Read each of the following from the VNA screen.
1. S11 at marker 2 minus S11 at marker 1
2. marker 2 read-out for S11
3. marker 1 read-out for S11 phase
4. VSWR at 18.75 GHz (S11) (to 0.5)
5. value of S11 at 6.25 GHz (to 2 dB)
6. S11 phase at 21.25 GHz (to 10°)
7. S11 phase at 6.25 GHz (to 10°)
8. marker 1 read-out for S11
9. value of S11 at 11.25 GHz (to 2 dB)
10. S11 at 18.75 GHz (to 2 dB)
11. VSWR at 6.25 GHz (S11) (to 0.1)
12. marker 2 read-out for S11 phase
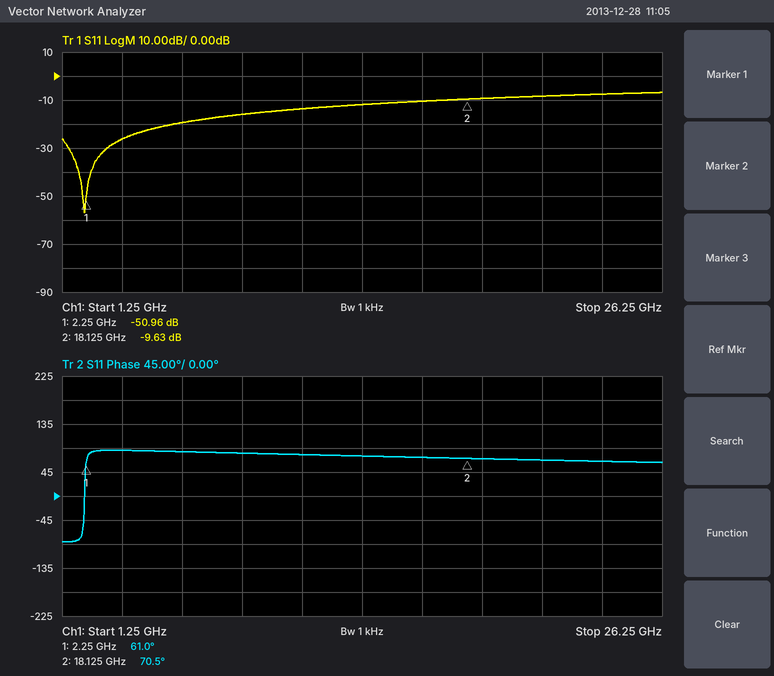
41.33 dB
-9.63 dB
61.0°
2.0
-20 dB
70°
80°
-50.96 dB
-14 dB
-10 dB
1.2
70.5°
